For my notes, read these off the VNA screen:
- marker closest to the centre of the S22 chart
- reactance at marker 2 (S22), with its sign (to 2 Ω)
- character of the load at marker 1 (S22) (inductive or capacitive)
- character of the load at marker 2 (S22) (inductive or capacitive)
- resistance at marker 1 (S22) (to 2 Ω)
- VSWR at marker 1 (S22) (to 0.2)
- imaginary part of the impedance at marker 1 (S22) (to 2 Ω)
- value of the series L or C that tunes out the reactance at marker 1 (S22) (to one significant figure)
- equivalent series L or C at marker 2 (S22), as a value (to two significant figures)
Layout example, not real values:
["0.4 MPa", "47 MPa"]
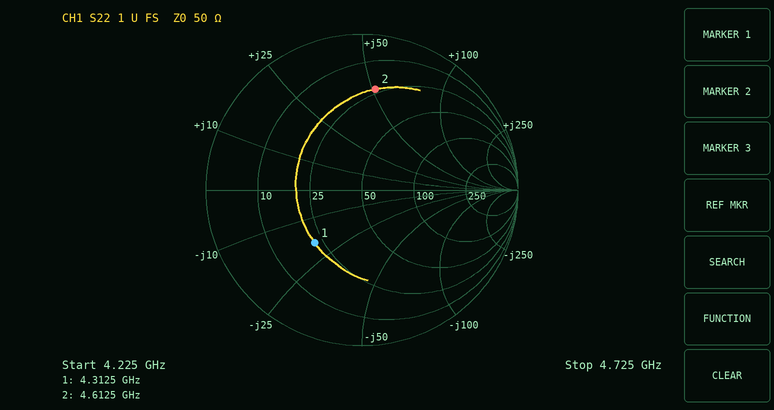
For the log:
["marker 1", "+52 Ω", "capacitive", "inductive", "22 Ω", "2.6", "-18 Ω", "700 pH", "1.8 nH"]
